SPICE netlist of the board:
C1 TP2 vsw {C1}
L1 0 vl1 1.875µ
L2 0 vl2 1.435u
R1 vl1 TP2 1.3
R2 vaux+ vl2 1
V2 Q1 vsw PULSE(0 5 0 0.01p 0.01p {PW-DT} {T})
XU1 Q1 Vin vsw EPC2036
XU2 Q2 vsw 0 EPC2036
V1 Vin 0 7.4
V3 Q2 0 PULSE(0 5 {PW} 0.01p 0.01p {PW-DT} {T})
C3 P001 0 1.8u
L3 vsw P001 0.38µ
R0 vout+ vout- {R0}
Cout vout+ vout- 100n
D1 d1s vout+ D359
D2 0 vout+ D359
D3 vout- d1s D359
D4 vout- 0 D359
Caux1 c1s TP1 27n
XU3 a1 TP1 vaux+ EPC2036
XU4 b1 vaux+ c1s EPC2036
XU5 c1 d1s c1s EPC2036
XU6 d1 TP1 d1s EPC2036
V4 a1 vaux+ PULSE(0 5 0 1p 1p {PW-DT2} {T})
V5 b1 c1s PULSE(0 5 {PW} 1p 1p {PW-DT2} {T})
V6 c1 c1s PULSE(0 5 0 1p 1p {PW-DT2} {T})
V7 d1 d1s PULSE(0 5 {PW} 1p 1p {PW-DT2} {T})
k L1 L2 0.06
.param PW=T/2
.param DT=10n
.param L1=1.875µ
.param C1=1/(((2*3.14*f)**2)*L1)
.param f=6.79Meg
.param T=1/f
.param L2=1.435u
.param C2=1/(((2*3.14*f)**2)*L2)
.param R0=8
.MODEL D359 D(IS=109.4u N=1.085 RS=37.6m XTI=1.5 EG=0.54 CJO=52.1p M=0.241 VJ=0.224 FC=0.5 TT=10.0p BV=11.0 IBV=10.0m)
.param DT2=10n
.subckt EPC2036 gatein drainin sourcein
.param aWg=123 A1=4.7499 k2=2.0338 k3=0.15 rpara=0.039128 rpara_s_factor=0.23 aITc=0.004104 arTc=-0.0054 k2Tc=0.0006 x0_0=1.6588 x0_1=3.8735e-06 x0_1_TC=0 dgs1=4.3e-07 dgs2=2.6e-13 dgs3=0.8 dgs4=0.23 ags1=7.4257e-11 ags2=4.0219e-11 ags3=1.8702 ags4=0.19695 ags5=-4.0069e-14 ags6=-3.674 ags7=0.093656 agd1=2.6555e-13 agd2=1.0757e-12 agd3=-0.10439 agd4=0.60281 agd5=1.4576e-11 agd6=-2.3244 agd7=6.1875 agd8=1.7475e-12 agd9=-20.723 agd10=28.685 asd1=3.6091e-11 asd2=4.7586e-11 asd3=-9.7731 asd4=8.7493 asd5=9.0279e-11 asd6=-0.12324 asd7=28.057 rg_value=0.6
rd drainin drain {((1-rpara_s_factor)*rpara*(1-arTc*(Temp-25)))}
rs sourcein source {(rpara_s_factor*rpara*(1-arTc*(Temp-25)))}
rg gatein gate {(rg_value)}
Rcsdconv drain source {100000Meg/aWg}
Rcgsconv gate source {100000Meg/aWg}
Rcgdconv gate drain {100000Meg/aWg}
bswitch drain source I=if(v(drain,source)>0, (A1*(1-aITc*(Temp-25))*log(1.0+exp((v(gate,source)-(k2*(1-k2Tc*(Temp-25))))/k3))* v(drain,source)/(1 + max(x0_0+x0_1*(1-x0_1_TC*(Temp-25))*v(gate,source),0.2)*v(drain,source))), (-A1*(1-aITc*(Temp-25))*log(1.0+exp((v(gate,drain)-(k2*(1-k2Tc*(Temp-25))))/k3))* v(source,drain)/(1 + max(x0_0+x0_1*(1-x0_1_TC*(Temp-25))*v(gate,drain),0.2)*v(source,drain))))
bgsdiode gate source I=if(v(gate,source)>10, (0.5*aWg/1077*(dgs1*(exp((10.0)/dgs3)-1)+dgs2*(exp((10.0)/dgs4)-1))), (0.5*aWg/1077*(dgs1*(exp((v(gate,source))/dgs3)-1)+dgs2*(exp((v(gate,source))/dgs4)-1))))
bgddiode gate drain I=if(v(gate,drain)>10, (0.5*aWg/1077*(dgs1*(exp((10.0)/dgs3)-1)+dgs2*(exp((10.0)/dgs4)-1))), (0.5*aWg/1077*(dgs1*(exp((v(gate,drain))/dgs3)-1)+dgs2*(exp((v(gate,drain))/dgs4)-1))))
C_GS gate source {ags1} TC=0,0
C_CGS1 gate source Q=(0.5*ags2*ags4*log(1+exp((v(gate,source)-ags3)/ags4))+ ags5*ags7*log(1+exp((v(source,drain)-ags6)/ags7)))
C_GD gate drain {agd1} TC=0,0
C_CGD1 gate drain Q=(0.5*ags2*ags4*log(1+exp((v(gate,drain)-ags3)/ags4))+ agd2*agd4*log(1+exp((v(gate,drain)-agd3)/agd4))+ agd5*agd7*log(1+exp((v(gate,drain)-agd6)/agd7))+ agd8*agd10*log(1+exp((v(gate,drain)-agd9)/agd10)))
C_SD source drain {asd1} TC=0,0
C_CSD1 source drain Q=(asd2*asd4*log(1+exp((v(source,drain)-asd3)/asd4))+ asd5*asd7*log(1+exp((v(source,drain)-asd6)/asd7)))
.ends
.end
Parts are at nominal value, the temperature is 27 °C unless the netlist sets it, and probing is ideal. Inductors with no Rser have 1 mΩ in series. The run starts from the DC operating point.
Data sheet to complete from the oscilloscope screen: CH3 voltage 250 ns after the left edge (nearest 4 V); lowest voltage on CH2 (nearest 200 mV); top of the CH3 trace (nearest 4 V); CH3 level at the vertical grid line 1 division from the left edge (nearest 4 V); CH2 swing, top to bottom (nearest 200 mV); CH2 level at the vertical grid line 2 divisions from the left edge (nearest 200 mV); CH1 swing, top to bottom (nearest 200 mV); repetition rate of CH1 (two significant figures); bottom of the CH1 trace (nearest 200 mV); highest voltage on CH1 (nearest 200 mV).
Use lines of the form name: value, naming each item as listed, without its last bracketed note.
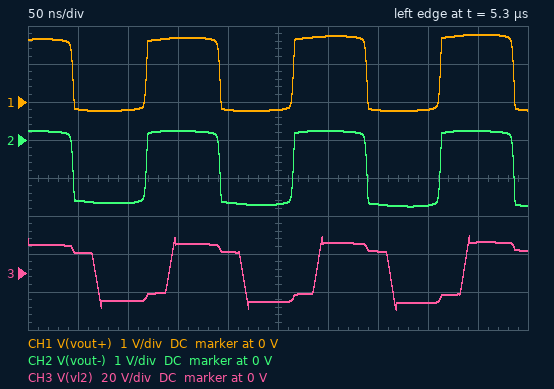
CH3 voltage 250 ns after the left edge: -16 V
lowest voltage on CH2: -1.8 V
top of the CH3 trace: 20 V
CH3 level at the vertical grid line 1 division from the left edge: 12 V
CH2 swing, top to bottom: 2.0 V
CH2 level at the vertical grid line 2 divisions from the left edge: -1.6 V
CH1 swing, top to bottom: 2.0 V
repetition rate of CH1: 6.8 MHz
bottom of the CH1 trace: -200 mV
highest voltage on CH1: 1.8 V
